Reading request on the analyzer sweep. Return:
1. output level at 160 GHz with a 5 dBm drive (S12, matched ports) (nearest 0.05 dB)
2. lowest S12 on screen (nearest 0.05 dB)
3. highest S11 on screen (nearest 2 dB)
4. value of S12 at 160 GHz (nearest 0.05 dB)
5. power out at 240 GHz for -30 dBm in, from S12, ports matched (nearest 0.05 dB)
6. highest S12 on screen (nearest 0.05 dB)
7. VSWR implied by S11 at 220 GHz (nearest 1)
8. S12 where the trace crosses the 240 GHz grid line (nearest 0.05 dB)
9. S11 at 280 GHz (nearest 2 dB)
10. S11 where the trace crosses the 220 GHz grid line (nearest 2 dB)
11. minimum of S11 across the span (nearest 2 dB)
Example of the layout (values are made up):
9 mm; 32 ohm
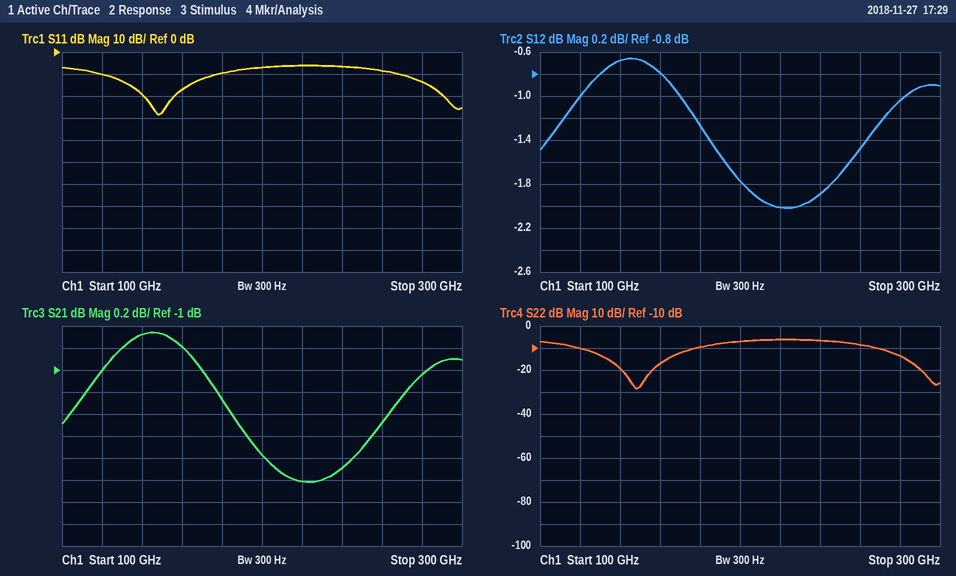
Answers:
4.20 dBm; -2.00 dB; -6 dB; -0.80 dB; -31.90 dBm; -0.65 dB; 3; -1.90 dB; -14 dB; -6 dB; -28 dB
